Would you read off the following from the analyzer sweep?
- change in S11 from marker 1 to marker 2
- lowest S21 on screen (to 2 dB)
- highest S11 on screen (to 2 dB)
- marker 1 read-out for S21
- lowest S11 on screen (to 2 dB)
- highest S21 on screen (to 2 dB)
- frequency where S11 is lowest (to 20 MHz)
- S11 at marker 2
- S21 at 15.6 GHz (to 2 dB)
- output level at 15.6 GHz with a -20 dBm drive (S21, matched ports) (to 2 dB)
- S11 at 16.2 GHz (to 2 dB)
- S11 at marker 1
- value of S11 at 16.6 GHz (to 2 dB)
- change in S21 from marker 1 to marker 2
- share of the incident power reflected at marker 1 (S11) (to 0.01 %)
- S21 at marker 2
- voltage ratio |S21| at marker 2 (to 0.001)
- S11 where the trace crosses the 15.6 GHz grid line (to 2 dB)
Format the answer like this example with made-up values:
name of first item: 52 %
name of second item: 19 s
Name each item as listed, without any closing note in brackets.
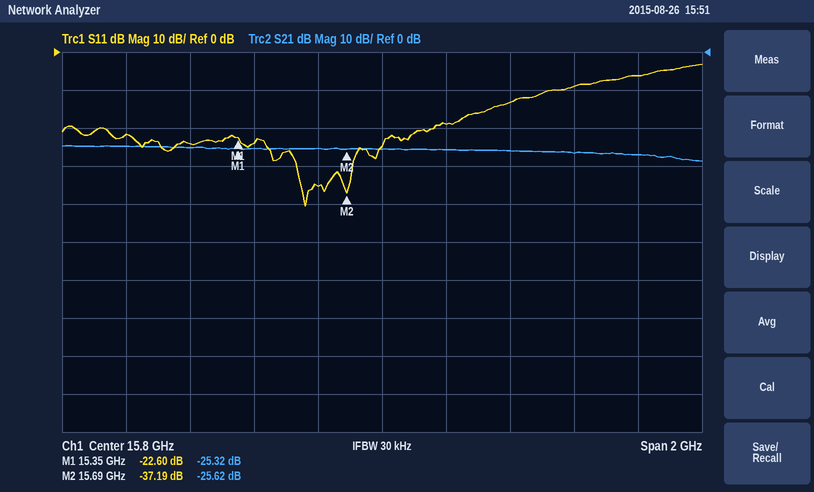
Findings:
change in S11 from marker 1 to marker 2: -14.59 dB
lowest S21 on screen: -28 dB
highest S11 on screen: -4 dB
marker 1 read-out for S21: -25.32 dB
lowest S11 on screen: -40 dB
highest S21 on screen: -24 dB
frequency where S11 is lowest: 15.56 GHz
S11 at marker 2: -37.19 dB
S21 at 15.6 GHz: -26 dB
output level at 15.6 GHz with a -20 dBm drive (S21, matched ports): -46 dBm
S11 at 16.2 GHz: -14 dB
S11 at marker 1: -22.60 dB
value of S11 at 16.6 GHz: -6 dB
change in S21 from marker 1 to marker 2: -0.30 dB
share of the incident power reflected at marker 1 (S11): 0.55 %
S21 at marker 2: -25.62 dB
voltage ratio |S21| at marker 2: 0.052
S11 where the trace crosses the 15.6 GHz grid line: -36 dB
